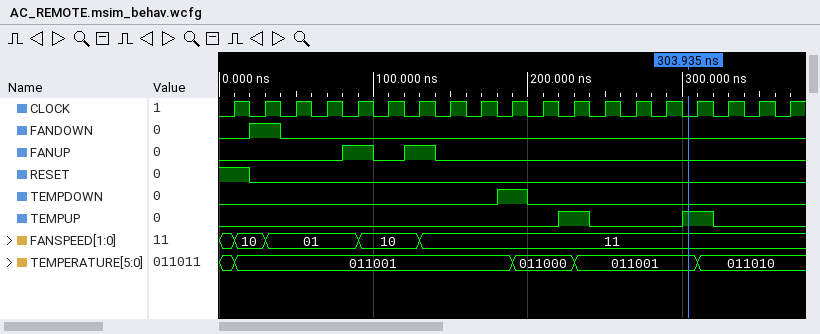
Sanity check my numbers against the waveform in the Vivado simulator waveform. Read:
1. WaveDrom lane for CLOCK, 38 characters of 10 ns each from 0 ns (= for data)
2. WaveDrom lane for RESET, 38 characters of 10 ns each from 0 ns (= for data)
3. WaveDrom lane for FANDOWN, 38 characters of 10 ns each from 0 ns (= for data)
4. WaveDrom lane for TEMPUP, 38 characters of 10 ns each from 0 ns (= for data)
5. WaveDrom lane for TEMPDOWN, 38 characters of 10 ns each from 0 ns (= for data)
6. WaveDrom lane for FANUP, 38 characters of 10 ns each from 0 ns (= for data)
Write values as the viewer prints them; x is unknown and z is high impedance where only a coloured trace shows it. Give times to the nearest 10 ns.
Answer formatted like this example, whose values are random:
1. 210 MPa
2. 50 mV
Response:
1. {name: 'CLOCK', wave: '01010101010101010101010101010101010101'}
2. {name: 'RESET', wave: '1.0...................................'}
3. {name: 'FANDOWN', wave: '0.1.0.................................'}
4. {name: 'TEMPUP', wave: '0.....................1.0.....1.0.....'}
5. {name: 'TEMPDOWN', wave: '0.................1.0.................'}
6. {name: 'FANUP', wave: '0.......1.0.1.0.......................'}
